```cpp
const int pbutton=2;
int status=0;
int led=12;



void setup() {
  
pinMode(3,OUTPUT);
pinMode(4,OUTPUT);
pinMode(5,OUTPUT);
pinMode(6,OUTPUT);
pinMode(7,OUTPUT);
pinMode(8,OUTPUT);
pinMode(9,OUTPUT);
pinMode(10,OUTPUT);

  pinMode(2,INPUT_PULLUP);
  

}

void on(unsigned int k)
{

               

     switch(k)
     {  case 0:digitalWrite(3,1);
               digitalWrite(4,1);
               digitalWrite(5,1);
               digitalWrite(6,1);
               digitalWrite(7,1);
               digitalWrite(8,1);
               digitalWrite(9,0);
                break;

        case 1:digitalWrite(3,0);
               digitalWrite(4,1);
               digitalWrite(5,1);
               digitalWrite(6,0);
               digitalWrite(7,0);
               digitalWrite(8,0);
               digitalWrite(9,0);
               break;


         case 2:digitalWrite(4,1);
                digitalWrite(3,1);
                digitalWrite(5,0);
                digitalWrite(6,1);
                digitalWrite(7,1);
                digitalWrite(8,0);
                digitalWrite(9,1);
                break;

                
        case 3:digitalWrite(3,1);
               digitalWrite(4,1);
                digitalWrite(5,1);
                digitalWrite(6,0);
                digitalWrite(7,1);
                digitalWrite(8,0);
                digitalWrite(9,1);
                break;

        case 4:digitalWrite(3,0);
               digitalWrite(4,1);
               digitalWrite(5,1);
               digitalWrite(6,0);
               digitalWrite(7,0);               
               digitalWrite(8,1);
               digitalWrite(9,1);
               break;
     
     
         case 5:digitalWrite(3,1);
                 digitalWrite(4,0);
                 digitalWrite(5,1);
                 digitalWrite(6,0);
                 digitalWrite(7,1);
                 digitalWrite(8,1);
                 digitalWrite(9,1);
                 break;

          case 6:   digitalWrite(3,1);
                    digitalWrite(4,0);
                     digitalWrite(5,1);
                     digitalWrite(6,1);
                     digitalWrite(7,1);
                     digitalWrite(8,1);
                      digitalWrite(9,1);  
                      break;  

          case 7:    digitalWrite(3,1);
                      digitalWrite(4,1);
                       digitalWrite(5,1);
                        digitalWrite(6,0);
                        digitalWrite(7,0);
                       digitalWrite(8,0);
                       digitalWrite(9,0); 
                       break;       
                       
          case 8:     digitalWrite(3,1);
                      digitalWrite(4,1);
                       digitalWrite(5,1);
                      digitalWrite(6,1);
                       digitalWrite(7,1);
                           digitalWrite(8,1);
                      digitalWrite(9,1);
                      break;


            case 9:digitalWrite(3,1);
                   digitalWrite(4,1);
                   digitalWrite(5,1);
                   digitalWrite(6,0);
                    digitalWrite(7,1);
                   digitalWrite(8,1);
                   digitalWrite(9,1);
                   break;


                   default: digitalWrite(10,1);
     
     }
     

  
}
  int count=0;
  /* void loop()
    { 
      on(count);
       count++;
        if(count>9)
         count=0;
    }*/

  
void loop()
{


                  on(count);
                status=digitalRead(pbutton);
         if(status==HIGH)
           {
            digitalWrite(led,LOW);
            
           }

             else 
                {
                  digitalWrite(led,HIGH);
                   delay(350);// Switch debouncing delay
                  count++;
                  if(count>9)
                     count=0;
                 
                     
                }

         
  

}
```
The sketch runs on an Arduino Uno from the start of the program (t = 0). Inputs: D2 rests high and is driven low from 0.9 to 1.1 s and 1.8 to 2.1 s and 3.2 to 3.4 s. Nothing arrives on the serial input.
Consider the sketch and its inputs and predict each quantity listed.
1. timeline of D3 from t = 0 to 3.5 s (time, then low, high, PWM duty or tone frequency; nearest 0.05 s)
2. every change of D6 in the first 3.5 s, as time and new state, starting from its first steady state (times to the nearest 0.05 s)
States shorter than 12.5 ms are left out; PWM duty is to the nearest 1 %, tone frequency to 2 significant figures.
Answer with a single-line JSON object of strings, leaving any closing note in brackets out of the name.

{"timeline of D3 from t = 0 to 3.5 s": "0 s high; 1.25 s low; 2.15 s high", "every change of D6 in the first 3.5 s, as time and new state, starting from its first steady state": "0 s high; 1.25 s low; 2.15 s high"}
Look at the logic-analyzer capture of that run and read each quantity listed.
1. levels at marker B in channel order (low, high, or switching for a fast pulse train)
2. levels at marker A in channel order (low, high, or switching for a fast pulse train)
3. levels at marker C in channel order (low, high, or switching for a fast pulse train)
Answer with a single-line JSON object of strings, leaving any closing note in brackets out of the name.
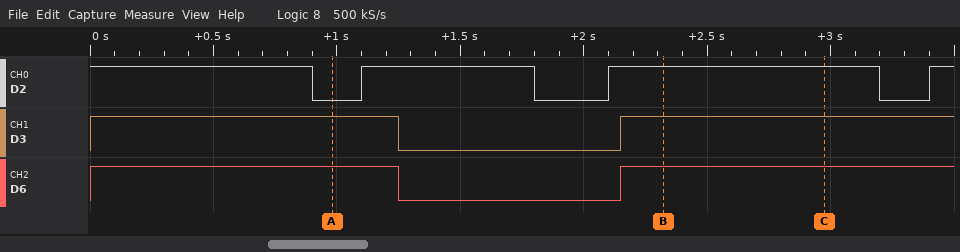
{"levels at marker B in channel order": "D2 high, D3 high, D6 high", "levels at marker A in channel order": "D2 low, D3 high, D6 high", "levels at marker C in channel order": "D2 high, D3 high, D6 high"}
